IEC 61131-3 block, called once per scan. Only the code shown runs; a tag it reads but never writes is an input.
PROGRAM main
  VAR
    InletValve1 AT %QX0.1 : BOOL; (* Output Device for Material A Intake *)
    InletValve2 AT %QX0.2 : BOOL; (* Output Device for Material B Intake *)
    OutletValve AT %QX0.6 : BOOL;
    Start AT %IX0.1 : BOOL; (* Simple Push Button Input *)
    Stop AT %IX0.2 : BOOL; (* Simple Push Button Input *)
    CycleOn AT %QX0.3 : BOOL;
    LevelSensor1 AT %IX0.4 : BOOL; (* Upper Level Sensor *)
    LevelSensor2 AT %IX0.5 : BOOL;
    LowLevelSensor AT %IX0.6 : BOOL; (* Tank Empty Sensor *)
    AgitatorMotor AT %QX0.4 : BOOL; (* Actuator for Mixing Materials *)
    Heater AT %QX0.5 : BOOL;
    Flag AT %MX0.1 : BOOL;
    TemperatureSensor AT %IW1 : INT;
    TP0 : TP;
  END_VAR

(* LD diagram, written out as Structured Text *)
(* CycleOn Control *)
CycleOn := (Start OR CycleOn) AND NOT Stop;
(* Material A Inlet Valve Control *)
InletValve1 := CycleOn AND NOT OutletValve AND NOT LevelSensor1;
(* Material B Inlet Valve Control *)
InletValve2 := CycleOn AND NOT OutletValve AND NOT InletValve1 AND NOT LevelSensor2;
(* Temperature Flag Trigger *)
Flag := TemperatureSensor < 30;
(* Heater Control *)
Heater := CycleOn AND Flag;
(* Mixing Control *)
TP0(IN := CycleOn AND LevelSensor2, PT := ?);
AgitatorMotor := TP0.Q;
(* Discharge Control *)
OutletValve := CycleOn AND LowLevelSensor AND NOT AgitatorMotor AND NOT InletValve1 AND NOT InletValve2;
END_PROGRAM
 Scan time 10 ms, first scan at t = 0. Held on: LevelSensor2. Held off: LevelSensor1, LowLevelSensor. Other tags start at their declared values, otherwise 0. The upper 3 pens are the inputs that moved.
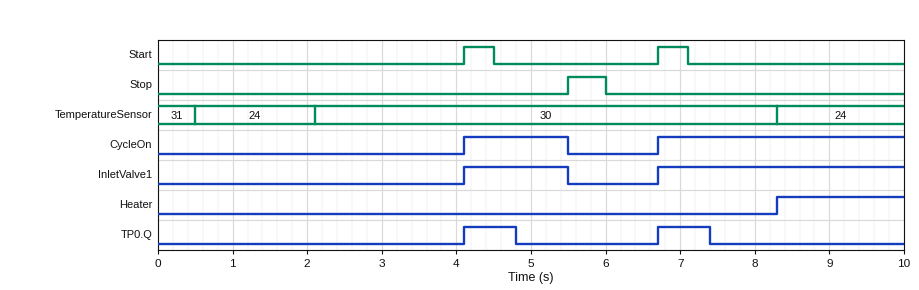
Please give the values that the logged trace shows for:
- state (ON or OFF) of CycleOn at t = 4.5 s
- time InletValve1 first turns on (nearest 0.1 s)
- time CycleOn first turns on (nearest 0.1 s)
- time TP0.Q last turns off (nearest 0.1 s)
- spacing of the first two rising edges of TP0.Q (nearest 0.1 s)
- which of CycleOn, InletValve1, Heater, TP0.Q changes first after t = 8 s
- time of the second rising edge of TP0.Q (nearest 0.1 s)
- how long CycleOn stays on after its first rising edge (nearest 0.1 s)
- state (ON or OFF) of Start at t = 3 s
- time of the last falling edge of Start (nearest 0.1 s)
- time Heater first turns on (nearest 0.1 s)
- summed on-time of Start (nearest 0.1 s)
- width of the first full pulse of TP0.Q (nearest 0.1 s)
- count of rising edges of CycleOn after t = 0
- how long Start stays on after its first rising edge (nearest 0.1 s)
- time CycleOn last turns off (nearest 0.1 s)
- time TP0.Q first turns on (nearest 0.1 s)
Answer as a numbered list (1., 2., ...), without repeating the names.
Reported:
1. ON
2. 4.1 s
3. 4.1 s
4. 7.4 s
5. 2.6 s
6. Heater
7. 6.7 s
8. 1.4 s
9. OFF
10. 7.1 s
11. 8.3 s
12. 0.8 s
13. 0.7 s
14. 2
15. 0.4 s
16. 5.5 s
17. 4.1 s
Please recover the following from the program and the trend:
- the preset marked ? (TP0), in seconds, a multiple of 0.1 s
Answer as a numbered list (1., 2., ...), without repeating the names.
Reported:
1. 0.7 s
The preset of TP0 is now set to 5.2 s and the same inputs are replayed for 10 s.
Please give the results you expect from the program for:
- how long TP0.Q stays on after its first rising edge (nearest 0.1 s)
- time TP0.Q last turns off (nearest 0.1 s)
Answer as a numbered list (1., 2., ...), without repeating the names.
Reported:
1. 5.2 s
2. 9.3 s
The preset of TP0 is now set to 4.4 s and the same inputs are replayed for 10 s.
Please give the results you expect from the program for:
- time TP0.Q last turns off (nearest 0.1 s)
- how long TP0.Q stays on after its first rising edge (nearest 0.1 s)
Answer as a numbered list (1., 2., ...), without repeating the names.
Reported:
1. 8.5 s
2. 4.4 s
